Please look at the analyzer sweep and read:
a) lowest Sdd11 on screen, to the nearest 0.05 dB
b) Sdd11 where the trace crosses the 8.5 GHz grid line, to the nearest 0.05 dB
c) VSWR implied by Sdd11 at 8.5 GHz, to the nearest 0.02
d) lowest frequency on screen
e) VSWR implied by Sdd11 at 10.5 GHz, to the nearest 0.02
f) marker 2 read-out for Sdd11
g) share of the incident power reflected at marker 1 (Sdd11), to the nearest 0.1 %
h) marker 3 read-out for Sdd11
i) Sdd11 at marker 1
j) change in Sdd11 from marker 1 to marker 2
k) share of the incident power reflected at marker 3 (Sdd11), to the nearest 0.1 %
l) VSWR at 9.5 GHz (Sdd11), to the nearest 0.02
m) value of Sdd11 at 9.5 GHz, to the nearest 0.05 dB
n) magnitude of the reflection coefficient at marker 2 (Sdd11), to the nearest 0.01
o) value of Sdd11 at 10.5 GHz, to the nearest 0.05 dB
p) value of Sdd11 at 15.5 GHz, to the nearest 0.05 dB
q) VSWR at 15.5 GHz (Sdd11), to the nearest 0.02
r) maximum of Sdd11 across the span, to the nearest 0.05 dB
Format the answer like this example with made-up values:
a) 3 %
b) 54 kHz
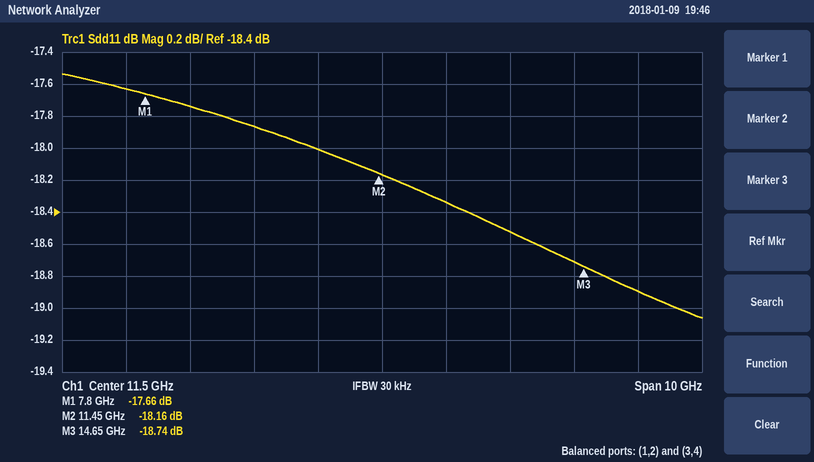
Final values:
a) -19.05 dB
b) -17.75 dB
c) 1.30
d) 6.5 GHz
e) 1.28
f) -18.16 dB
g) 1.7 %
h) -18.74 dB
i) -17.66 dB
j) -0.50 dB
k) 1.3 %
l) 1.30
m) -17.85 dB
n) 0.12
o) -18.00 dB
p) -18.90 dB
q) 1.26
r) -17.55 dB
